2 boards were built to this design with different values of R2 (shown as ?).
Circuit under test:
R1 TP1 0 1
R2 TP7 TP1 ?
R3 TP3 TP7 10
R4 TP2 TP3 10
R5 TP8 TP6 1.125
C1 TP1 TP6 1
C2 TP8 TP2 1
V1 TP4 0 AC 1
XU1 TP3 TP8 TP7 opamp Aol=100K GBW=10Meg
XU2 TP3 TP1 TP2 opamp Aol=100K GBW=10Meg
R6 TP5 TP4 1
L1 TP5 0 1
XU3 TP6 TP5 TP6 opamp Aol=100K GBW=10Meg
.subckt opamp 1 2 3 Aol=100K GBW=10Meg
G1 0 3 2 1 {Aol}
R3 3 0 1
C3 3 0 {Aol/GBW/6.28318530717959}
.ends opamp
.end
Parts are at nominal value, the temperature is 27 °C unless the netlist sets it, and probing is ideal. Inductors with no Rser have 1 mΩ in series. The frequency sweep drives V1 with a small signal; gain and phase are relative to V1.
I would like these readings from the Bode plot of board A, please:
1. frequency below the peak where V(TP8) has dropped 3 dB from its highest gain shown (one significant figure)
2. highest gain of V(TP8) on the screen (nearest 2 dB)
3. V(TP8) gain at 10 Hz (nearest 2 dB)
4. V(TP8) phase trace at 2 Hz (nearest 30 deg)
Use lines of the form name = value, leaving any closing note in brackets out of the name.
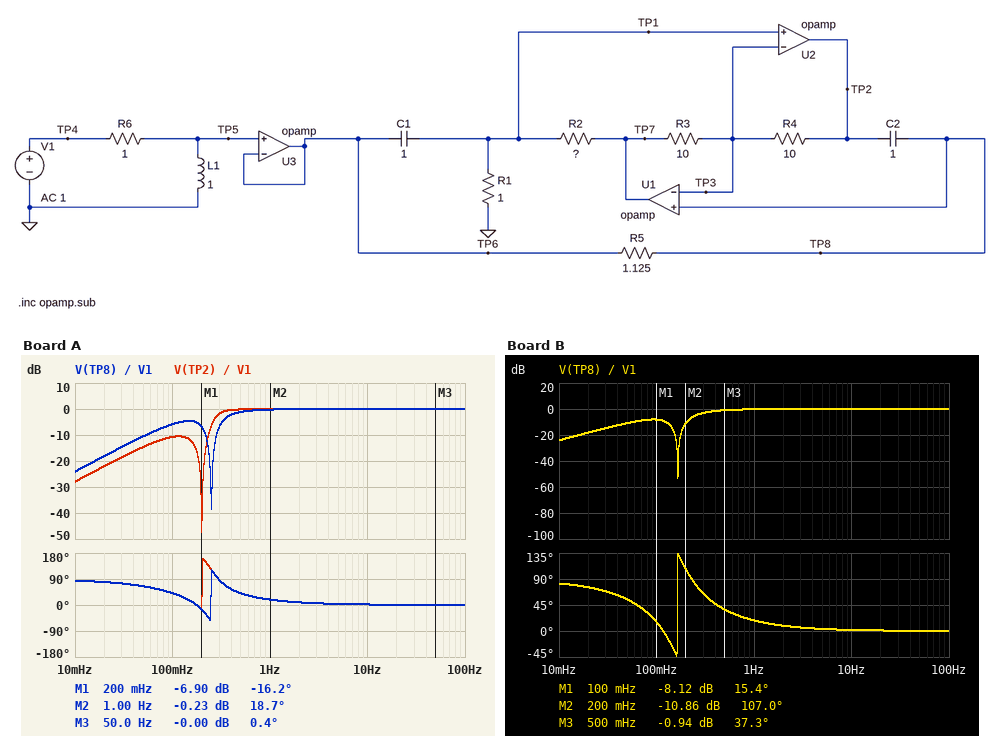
frequency below the peak where V(TP8) has dropped 3 dB from its highest gain shown = 400 mHz
highest gain of V(TP8) on the screen = 0 dB
V(TP8) gain at 10 Hz = 0 dB
V(TP8) phase trace at 2 Hz = 0 deg
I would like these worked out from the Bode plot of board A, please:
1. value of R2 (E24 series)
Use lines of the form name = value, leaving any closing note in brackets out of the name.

value of R2 = 0.36 Ω
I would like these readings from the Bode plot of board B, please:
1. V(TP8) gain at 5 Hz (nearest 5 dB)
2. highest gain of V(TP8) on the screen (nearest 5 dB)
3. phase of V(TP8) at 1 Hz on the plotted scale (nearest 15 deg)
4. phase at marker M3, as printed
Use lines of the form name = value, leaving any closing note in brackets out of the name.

V(TP8) gain at 5 Hz = 0 dB
highest gain of V(TP8) on the screen = 0 dB
phase of V(TP8) at 1 Hz on the plotted scale = 15 deg
phase at marker M3, as printed = 37.3 deg
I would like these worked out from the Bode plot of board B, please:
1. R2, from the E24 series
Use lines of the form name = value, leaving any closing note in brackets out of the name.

R2, from the E24 series = 0.82 Ω
